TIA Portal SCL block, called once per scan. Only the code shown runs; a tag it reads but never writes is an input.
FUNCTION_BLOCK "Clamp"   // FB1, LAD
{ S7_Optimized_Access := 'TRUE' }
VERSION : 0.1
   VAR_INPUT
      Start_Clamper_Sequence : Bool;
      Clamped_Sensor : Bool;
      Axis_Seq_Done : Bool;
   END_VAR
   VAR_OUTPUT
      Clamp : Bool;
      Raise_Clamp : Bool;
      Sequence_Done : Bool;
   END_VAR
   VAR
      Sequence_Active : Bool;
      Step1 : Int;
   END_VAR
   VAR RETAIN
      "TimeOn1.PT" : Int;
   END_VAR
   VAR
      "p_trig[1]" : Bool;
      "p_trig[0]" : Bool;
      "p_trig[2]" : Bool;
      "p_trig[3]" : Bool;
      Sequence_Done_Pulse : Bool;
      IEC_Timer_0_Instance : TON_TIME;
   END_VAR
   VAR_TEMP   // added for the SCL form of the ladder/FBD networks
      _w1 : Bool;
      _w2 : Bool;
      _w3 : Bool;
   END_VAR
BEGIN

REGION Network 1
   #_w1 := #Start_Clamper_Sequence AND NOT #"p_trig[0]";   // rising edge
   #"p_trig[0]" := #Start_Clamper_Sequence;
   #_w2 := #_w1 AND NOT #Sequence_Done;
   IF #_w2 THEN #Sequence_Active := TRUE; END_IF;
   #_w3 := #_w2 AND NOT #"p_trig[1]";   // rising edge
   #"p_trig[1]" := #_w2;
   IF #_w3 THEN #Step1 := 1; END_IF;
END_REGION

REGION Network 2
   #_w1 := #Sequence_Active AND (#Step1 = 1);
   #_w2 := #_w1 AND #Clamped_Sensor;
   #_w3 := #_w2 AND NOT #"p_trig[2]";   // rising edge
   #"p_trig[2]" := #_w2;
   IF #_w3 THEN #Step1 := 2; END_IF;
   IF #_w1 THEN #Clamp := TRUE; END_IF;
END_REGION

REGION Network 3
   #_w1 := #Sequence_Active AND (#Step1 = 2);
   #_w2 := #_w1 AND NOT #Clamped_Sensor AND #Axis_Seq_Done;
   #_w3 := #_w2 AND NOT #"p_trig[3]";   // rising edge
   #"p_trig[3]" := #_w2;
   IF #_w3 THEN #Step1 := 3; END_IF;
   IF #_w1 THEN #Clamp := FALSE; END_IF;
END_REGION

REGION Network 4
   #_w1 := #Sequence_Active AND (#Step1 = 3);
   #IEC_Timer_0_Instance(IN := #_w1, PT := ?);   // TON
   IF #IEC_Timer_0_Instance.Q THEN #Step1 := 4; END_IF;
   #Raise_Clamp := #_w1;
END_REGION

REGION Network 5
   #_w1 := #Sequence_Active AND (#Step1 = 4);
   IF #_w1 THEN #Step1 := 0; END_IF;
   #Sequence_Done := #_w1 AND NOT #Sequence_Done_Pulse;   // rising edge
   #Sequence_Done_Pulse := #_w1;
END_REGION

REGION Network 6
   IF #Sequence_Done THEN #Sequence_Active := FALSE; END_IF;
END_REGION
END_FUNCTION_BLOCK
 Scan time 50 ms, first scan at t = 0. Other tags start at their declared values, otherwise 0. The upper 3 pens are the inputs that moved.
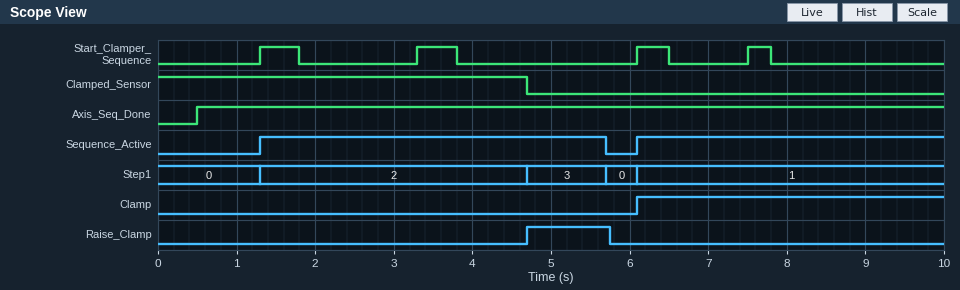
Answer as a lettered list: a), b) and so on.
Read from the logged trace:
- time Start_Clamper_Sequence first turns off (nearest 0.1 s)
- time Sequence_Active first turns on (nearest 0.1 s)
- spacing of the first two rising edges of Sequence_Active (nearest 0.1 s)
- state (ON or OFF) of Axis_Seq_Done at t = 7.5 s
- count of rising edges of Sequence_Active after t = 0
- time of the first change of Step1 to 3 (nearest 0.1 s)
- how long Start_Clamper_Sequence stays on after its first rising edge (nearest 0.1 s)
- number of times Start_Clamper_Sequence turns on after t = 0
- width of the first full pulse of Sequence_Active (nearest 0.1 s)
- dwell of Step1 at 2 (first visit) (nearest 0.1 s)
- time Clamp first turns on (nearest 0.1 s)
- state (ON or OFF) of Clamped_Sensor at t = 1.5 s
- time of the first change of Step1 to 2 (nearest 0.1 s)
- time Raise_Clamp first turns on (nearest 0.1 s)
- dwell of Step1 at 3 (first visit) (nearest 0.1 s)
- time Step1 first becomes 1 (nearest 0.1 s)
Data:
a) 1.8 s
b) 1.3 s
c) 4.8 s
d) ON
e) 2
f) 4.7 s
g) 0.5 s
h) 4
i) 4.4 s
j) 3.4 s
k) 6.1 s
l) ON
m) 1.3 s
n) 4.7 s
o) 1.0 s
p) 6.1 s
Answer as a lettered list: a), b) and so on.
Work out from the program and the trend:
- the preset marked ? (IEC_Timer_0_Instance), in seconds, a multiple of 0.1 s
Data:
a) 1.0 s
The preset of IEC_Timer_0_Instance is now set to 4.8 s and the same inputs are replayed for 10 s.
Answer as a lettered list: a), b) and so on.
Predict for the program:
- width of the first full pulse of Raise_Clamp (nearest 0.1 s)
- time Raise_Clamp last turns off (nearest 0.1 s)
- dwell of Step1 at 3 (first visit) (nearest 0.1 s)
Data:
a) 1.4 s
b) 6.1 s
c) 1.4 s
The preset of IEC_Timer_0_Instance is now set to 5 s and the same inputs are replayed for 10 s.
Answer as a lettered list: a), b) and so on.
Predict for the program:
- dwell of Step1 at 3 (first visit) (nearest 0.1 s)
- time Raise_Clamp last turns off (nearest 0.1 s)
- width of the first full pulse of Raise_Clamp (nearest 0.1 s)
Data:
a) 1.4 s
b) 6.1 s
c) 1.4 s
